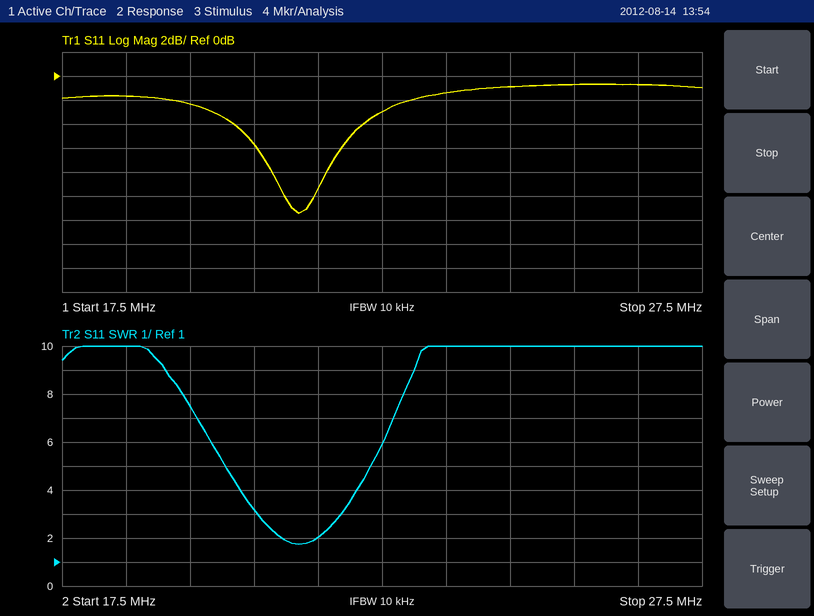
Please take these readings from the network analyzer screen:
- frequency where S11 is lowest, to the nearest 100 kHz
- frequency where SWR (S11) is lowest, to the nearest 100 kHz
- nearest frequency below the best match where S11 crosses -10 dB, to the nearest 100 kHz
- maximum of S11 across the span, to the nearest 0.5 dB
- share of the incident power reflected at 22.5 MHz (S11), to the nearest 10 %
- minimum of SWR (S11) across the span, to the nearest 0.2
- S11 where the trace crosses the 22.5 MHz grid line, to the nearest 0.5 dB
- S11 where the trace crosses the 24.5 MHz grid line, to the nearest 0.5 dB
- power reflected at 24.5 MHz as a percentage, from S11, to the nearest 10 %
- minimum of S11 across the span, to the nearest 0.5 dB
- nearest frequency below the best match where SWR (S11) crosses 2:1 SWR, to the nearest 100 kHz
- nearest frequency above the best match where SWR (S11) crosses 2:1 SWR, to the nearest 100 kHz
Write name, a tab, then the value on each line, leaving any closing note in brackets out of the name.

frequency where S11 is lowest, to the nearest 100 kHz	21.2 MHz
frequency where SWR (S11) is lowest, to the nearest 100 kHz	21.2 MHz
nearest frequency below the best match where S11 crosses -10 dB, to the nearest 100 kHz	21.0 MHz
maximum of S11 across the span, to the nearest 0.5 dB	-0.5 dB
share of the incident power reflected at 22.5 MHz (S11), to the nearest 10 %	50 %
minimum of SWR (S11) across the span, to the nearest 0.2	1.8
S11 where the trace crosses the 22.5 MHz grid line, to the nearest 0.5 dB	-3.0 dB
S11 where the trace crosses the 24.5 MHz grid line, to the nearest 0.5 dB	-1.0 dB
power reflected at 24.5 MHz as a percentage, from S11, to the nearest 10 %	80 %
minimum of S11 across the span, to the nearest 0.5 dB	-11.5 dB
nearest frequency below the best match where SWR (S11) crosses 2:1 SWR, to the nearest 100 kHz	20.9 MHz
nearest frequency above the best match where SWR (S11) crosses 2:1 SWR, to the nearest 100 kHz	21.5 MHz
